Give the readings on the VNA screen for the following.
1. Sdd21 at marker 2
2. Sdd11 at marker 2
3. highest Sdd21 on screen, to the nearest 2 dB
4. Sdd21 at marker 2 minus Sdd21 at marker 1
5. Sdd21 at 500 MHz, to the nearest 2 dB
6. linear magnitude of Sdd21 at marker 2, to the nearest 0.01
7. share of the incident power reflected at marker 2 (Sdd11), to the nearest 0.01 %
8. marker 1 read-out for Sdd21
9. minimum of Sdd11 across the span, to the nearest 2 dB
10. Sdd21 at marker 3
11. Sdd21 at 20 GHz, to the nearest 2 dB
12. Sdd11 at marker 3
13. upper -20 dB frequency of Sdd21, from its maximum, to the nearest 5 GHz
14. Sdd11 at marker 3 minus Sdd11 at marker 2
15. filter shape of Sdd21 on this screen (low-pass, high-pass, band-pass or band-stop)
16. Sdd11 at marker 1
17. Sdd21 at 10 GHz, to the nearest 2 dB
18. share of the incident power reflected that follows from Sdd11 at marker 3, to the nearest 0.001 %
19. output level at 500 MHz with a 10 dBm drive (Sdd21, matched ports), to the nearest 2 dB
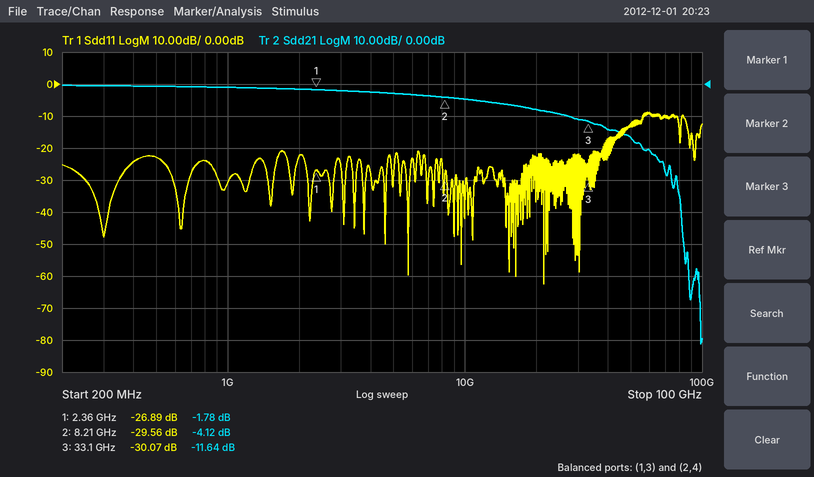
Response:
-4.12 dB
-29.56 dB
0 dB
-2.34 dB
0 dB
0.62
0.11 %
-1.78 dB
-62 dB
-11.64 dB
-8 dB
-30.07 dB
55 GHz
-0.51 dB
low-pass
-26.89 dB
-4 dB
0.098 %
10 dBm
